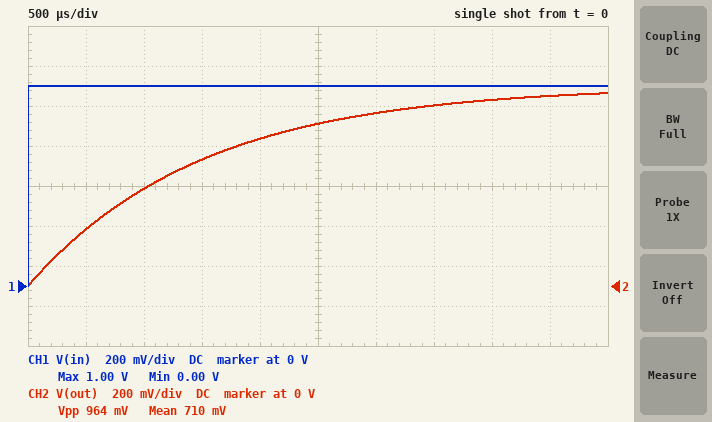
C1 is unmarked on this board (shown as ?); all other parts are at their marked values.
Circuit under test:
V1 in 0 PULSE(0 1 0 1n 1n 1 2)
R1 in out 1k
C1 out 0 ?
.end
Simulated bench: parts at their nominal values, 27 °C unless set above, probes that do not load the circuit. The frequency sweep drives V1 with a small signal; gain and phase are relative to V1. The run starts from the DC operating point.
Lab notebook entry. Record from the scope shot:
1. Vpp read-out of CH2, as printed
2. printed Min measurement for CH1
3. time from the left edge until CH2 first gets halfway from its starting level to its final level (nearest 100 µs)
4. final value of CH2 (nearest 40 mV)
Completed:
964 mV
0.00 V
1.0 ms
960 mV
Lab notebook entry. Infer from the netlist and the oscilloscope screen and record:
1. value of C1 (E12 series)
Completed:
1.5 µF
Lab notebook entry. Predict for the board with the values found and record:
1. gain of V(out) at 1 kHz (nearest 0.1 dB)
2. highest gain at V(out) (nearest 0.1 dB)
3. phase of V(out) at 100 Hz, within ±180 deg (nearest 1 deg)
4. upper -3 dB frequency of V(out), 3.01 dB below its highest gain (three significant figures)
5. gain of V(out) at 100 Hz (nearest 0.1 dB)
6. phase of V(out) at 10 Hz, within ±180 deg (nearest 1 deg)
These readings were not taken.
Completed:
-19.5 dB
0 dB
-43 deg
106 Hz
-2.8 dB
-5 deg
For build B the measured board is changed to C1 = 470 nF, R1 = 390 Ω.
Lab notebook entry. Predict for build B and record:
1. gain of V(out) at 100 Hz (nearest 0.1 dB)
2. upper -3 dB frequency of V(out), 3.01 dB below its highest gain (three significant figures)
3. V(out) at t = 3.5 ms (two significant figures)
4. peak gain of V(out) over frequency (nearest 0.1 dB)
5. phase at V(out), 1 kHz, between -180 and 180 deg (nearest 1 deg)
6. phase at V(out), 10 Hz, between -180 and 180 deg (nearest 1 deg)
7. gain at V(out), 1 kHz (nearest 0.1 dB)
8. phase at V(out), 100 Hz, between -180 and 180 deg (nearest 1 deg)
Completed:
-0.1 dB
868 Hz
1.0 V
0 dB
-49 deg
-1 deg
-3.7 dB
-7 deg
